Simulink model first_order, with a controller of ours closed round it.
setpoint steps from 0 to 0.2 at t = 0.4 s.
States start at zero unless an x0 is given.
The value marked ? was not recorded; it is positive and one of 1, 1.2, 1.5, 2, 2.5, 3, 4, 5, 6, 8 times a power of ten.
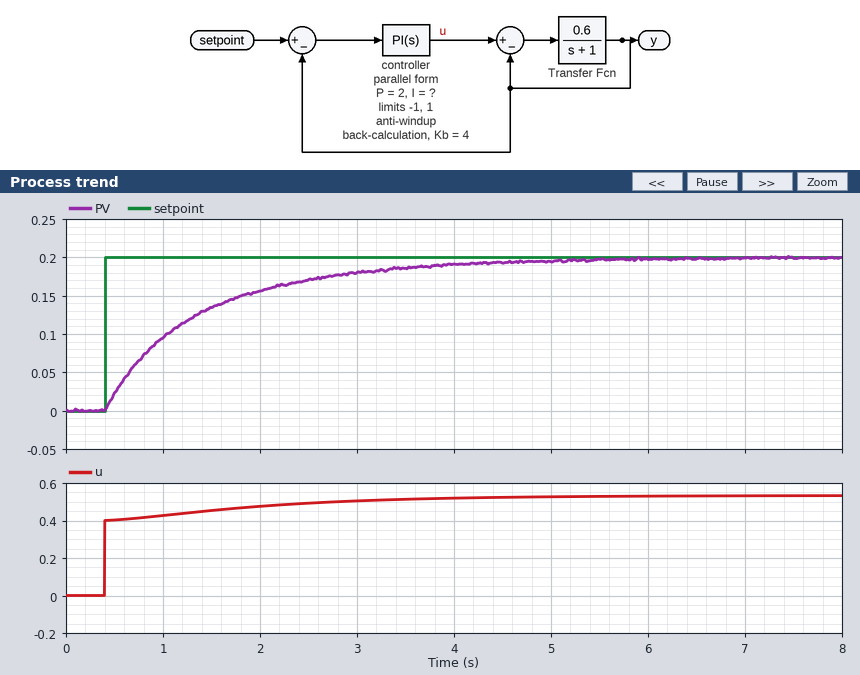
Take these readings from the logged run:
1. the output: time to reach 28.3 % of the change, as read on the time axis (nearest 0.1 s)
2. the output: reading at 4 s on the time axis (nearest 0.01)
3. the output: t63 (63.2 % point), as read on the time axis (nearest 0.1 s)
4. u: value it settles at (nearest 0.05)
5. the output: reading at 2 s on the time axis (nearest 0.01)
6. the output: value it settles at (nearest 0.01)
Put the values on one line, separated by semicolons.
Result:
0.7 s; 0.19; 1.4 s; 0.55; 0.16; 0.20
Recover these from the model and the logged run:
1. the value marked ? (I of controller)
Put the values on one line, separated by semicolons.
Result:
2.5
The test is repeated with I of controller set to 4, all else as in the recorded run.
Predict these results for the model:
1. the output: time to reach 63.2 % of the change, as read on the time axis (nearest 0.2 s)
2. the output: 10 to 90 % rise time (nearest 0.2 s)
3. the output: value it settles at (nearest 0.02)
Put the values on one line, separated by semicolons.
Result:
1.2 s; 1.4 s; 0.20
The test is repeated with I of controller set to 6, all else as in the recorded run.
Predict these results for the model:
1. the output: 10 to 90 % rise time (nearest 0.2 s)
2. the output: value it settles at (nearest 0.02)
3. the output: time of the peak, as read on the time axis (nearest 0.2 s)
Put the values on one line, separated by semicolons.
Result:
1.0 s; 0.20; 2.4 s
